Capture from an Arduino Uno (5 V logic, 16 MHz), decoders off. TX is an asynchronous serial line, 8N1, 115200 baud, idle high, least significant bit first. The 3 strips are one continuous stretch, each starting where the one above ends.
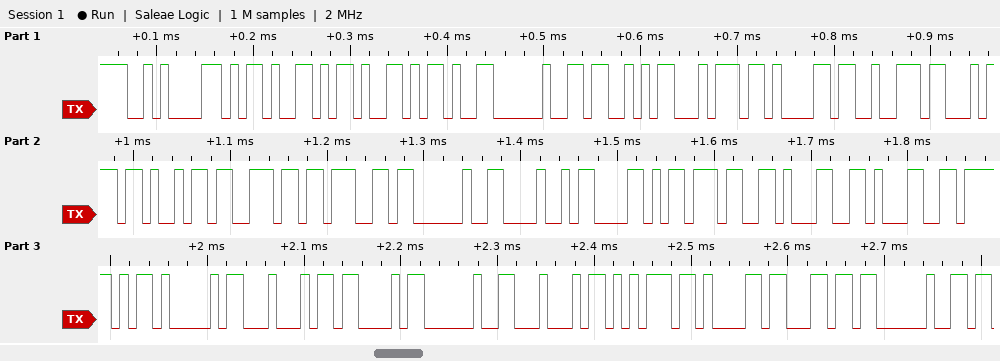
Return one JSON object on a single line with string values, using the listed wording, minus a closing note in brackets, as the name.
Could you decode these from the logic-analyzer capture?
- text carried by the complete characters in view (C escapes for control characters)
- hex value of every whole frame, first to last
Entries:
{"text carried by the complete characters in view": "\"\\n--- Starting HX711_ADC Dual \"", "hex value of every whole frame, first to last": "0x0A 0x2D 0x2D 0x2D 0x20 0x53 0x74 0x61 0x72 0x74 0x69 0x6E 0x67 0x20 0x48 0x58 0x37 0x31 0x31 0x5F 0x41 0x44 0x43 0x20 0x44 0x75 0x61 0x6C 0x20"}
